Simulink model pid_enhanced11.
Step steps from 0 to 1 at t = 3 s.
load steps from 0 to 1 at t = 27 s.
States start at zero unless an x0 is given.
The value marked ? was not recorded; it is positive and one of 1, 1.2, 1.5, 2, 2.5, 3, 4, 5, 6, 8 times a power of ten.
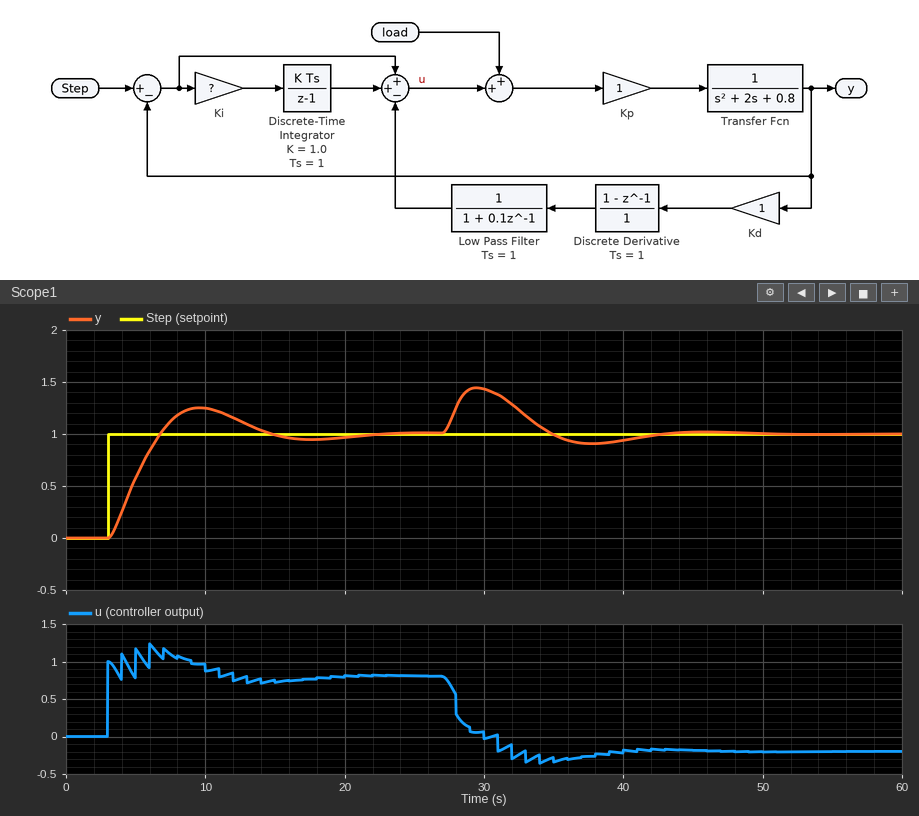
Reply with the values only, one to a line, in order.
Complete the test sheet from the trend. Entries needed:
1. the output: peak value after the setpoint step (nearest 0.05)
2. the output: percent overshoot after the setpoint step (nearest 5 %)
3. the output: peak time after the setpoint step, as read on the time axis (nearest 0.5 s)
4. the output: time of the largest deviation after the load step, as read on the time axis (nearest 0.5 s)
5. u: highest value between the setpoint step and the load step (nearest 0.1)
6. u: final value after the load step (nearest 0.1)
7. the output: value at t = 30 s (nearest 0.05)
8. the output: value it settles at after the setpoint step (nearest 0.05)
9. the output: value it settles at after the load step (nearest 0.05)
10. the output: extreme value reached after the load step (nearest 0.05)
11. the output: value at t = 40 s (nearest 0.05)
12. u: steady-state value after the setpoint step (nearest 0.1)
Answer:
1.25
25 %
9.5 s
29.5 s
1.2
-0.2
1.45
1.00
1.00
1.45
0.95
0.8
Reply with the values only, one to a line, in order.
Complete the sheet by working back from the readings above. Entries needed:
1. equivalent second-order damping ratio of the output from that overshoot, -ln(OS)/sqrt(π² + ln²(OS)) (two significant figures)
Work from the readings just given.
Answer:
0.40
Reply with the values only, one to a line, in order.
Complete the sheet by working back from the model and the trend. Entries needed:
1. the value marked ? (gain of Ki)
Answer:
0.6
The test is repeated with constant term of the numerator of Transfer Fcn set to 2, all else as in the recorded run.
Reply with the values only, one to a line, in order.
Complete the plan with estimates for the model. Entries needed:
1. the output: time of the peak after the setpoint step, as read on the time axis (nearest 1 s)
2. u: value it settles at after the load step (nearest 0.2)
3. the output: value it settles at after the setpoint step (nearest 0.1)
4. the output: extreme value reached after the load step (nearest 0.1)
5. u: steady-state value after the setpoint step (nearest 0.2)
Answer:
8 s
-0.6
1.0
1.6
0.4
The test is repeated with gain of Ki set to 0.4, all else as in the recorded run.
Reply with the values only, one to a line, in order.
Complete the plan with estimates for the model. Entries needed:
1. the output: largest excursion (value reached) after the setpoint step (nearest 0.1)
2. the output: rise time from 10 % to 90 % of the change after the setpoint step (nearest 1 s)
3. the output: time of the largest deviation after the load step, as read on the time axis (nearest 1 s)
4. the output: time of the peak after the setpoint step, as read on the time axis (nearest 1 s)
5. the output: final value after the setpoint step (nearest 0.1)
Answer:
1.1
4 s
30 s
11 s
1.0
